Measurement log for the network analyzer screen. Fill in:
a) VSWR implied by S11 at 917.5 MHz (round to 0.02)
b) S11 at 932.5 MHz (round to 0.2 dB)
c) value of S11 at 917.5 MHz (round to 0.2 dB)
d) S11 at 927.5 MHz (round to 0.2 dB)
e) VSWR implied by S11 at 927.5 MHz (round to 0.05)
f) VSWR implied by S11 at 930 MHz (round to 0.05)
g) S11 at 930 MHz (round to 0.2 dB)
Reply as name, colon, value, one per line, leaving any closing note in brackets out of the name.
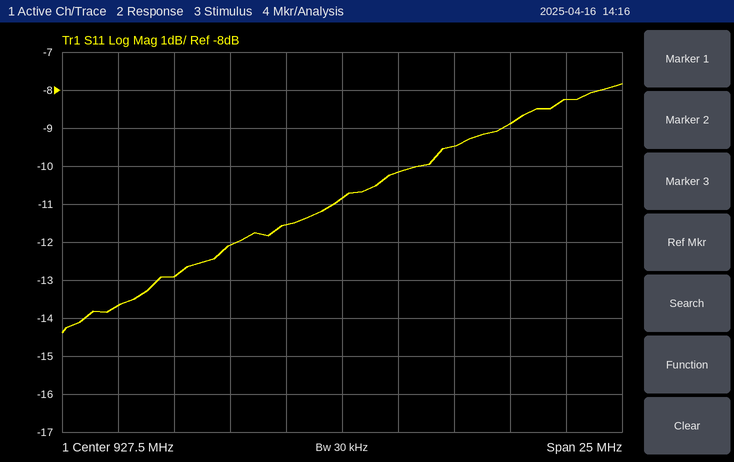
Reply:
VSWR implied by S11 at 917.5 MHz: 1.52
S11 at 932.5 MHz: -9.4 dB
value of S11 at 917.5 MHz: -13.6 dB
S11 at 927.5 MHz: -10.8 dB
VSWR implied by S11 at 927.5 MHz: 1.80
VSWR implied by S11 at 930 MHz: 1.90
S11 at 930 MHz: -10.2 dB
